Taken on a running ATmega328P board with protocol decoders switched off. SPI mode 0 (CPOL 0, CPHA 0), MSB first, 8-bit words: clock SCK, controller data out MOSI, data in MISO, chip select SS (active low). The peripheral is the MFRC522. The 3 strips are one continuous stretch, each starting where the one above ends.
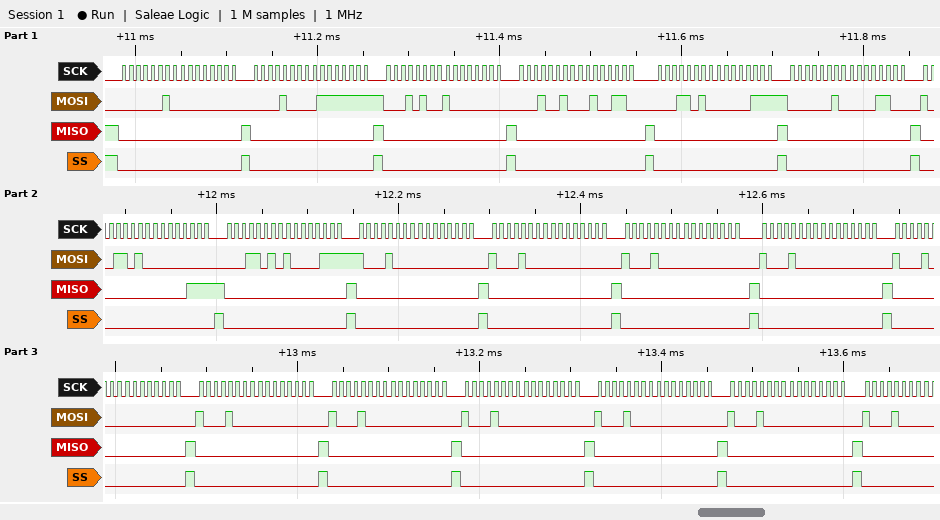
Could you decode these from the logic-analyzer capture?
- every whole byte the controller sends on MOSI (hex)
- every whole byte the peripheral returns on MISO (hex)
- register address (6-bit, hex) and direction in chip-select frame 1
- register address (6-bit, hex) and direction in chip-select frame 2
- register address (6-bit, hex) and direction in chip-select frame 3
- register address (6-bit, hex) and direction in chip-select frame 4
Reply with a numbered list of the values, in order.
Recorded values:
1. 02 00 08 7F 14 80 12 26 1A 07 02 0C 9A 00 1A 87 88 00 88 00 88 00 88 00 88 00 88 00 88 00 88 00 88 00 88 00 88
2. 00 00 00 00 00 00 00 00 00 00 00 00 00 07 00 00 00 00 00 00 00 00 00 00 00 00 00 00 00 00 00 00 00 00 00 00 00
3. 0x01 write
4. 0x04 write
5. 0x0A write
6. 0x09 write
